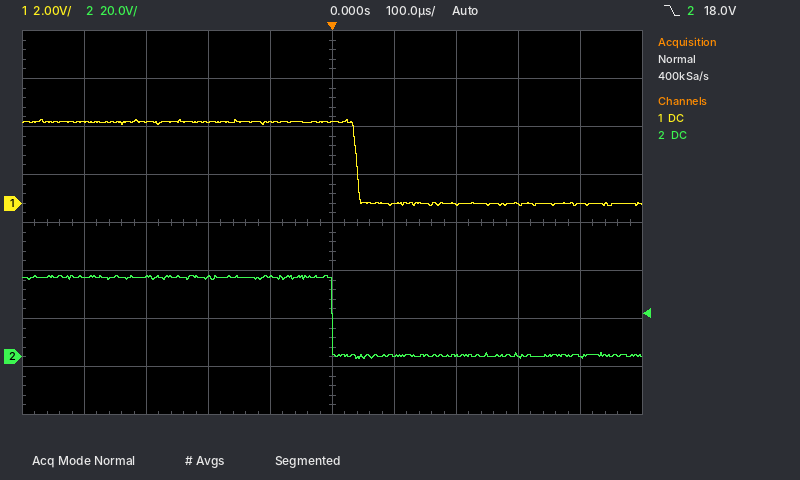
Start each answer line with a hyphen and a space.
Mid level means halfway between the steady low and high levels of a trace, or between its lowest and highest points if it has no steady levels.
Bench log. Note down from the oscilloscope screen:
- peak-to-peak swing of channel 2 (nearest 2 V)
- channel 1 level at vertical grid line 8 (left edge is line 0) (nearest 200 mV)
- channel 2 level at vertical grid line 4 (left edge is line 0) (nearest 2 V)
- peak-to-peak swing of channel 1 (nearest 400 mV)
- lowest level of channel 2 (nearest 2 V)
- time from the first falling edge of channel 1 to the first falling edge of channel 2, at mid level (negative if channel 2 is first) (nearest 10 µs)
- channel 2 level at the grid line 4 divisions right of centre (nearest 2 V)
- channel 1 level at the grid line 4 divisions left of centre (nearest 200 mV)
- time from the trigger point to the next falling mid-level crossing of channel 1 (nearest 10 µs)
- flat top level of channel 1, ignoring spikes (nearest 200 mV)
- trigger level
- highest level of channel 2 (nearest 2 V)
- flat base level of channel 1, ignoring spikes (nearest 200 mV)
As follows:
- 34 V
- 0.0 V
- 34 V
- 3.6 V
- 0 V
- -40 µs
- 0 V
- 3.4 V
- 40 µs
- 3.4 V
- 18.0 V
- 34 V
- 0.0 V
